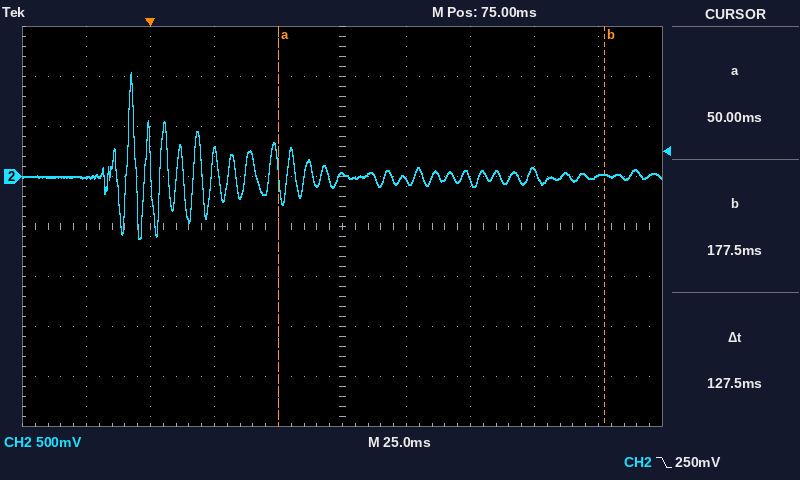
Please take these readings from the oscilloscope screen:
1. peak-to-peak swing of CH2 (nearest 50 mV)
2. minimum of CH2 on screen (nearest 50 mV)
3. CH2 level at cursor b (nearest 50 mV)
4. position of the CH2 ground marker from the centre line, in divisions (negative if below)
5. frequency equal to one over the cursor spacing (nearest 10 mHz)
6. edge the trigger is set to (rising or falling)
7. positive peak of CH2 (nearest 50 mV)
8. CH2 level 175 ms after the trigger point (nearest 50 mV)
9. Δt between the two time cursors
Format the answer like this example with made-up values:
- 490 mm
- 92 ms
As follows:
- 1.65 V
- -600 mV
- 0 mV
- +1.0 div
- 7.84 Hz
- falling
- 1.05 V
- 0 mV
- 127.5 ms
